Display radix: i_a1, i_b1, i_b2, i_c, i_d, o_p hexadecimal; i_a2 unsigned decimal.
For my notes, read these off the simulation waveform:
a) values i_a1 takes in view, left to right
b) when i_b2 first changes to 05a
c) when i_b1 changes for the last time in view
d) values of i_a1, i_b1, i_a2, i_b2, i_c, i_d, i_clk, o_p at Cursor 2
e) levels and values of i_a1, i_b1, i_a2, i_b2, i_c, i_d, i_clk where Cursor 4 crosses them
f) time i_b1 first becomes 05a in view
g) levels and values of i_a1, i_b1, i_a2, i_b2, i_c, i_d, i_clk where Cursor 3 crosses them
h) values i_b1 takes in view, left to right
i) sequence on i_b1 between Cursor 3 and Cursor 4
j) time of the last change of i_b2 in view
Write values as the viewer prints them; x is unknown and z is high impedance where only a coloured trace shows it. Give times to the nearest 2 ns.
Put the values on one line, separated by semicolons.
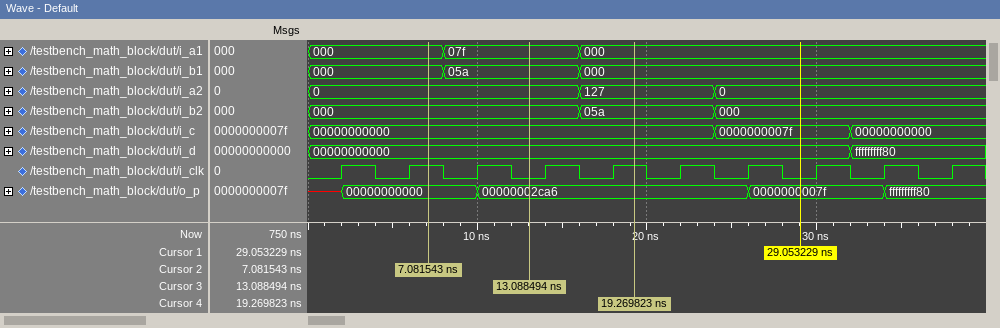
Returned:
000, 07f, 000; 16 ns; 16 ns; i_a1=000, i_b1=000, i_a2=0, i_b2=000, i_c=00000000000, i_d=00000000000, i_clk=1, o_p=00000000000; i_a1=000, i_b1=000, i_a2=127, i_b2=05a, i_c=00000000000, i_d=00000000000, i_clk=1; 8 ns; i_a1=07f, i_b1=05a, i_a2=0, i_b2=000, i_c=00000000000, i_d=00000000000, i_clk=0; 000, 05a, 000; 05a, 000; 24 ns
